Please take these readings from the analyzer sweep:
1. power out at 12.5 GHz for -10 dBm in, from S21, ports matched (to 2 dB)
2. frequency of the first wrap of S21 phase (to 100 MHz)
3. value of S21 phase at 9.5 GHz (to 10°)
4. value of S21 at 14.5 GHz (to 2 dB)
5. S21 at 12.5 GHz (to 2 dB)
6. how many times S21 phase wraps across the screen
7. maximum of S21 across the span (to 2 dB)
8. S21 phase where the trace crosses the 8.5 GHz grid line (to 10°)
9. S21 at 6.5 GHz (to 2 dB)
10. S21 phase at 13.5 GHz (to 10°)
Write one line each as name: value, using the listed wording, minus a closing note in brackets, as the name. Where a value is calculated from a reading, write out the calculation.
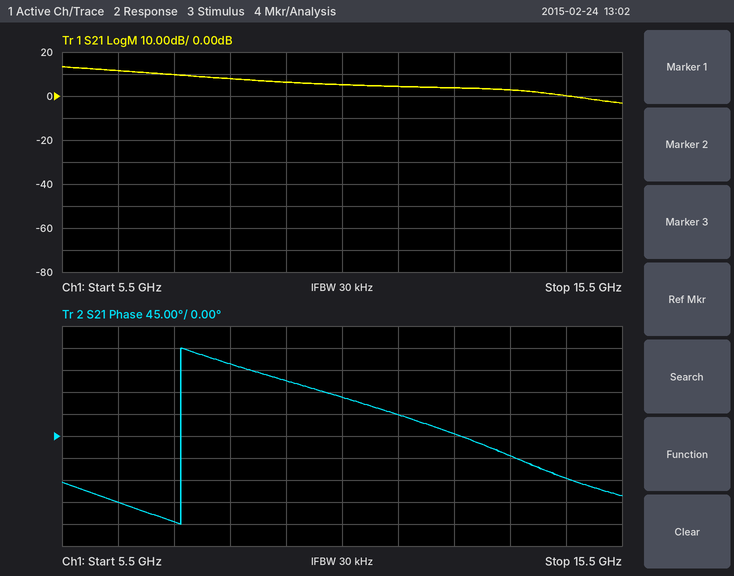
power out at 12.5 GHz for -10 dBm in, from S21, ports matched: -10 dBm + (4 dB) = -6 dBm
frequency of the first wrap of S21 phase: 7.6 GHz
value of S21 phase at 9.5 GHz: 110°
value of S21 at 14.5 GHz: 0 dB
S21 at 12.5 GHz: 4 dB
how many times S21 phase wraps across the screen: 1
maximum of S21 across the span: 14 dB
S21 phase where the trace crosses the 8.5 GHz grid line: 150°
S21 at 6.5 GHz: 12 dB
S21 phase at 13.5 GHz: -40°
